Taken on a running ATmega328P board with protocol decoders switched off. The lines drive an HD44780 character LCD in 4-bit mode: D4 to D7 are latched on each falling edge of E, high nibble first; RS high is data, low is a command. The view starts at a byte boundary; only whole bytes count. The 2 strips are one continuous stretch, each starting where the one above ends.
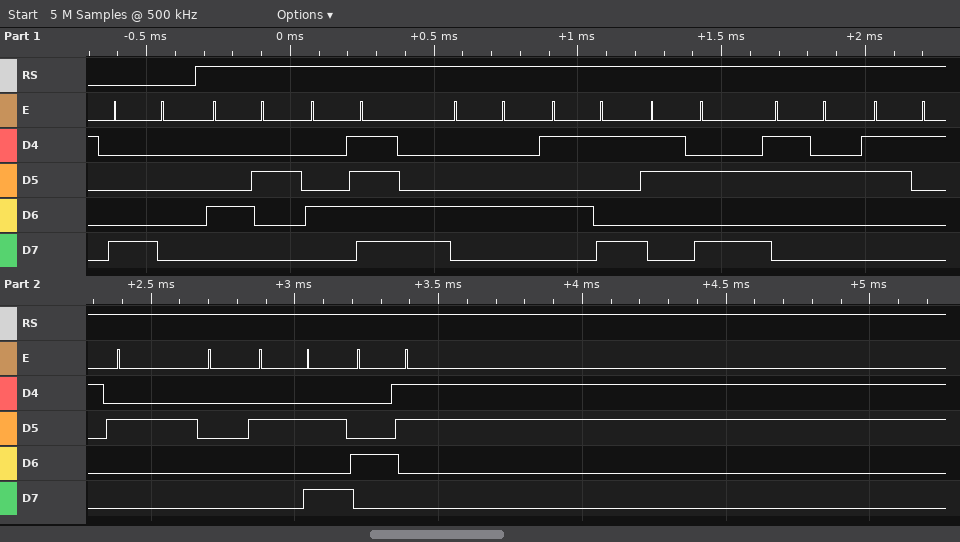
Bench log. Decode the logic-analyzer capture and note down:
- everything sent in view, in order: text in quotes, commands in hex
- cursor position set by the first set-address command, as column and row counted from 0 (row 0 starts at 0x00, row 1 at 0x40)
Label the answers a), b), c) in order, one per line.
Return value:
a) 0x80 "BODY:21 *C"
b) column 0, row 0
